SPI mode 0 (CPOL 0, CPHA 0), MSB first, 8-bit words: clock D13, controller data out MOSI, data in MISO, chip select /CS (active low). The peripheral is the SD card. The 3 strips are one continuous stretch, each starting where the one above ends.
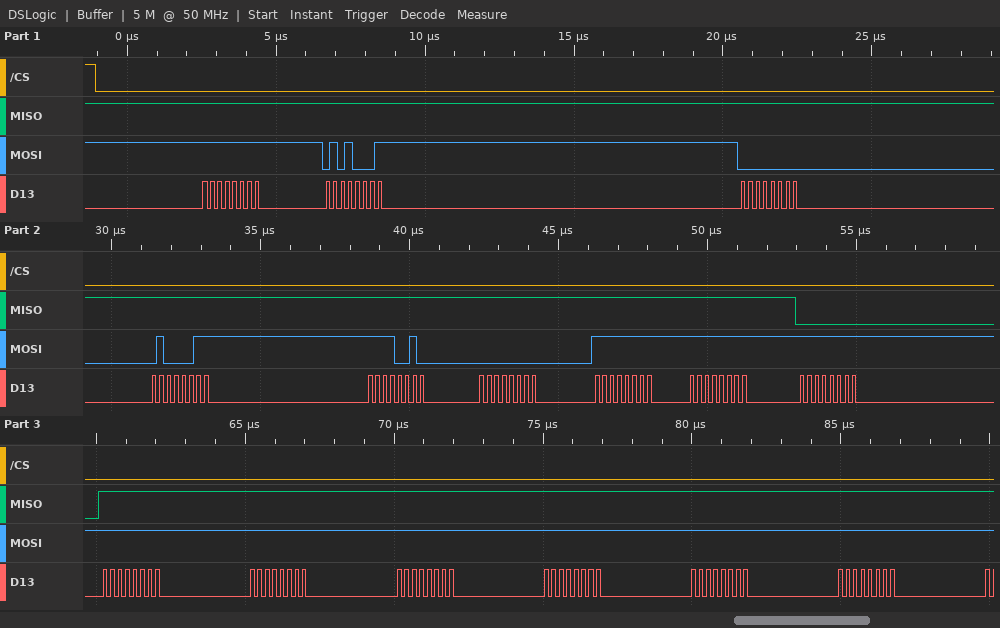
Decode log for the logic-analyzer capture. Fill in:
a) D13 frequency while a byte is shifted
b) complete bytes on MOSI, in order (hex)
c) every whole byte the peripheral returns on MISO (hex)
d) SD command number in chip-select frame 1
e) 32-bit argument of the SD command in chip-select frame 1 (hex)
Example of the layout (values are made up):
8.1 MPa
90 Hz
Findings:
4 MHz
FF 51 00 43 F2 00 FF FF FF FF FF FF FF FF FF
FF FF FF FF FF FF FF FF 00 FF FF FF FF FF FF
CMD17
0x0043F200
